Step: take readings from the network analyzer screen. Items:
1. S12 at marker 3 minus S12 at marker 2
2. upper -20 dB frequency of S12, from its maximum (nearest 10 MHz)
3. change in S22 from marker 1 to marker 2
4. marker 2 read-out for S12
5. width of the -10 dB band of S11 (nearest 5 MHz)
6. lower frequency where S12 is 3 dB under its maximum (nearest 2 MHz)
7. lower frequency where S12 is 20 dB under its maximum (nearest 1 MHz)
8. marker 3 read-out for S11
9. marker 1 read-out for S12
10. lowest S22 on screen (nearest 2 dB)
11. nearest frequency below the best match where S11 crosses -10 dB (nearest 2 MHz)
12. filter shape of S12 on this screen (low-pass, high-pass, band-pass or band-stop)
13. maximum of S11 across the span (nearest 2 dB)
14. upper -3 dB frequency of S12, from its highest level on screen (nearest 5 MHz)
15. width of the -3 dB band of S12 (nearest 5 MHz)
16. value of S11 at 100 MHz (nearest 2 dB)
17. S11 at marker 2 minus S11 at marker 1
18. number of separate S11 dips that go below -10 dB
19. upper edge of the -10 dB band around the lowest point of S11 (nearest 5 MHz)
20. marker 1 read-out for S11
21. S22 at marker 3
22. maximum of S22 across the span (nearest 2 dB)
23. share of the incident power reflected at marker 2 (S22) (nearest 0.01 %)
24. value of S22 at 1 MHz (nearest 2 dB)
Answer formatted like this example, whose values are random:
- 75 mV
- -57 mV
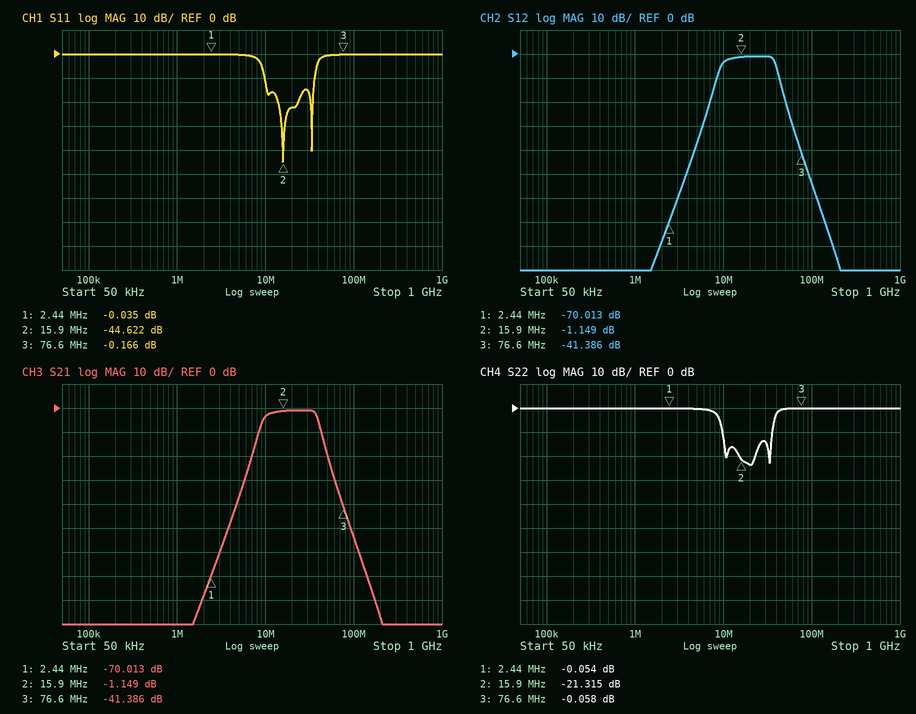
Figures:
- -40.237 dB
- 50 MHz
- -21.261 dB
- -1.149 dB
- 25 MHz
- 10 MHz
- 7 MHz
- -0.166 dB
- -70.013 dB
- -24 dB
- 10 MHz
- band-pass
- 0 dB
- 40 MHz
- 30 MHz
- 0 dB
- -44.587 dB
- 2
- 35 MHz
- -0.035 dB
- -0.058 dB
- 0 dB
- 0.74 %
- 0 dB
